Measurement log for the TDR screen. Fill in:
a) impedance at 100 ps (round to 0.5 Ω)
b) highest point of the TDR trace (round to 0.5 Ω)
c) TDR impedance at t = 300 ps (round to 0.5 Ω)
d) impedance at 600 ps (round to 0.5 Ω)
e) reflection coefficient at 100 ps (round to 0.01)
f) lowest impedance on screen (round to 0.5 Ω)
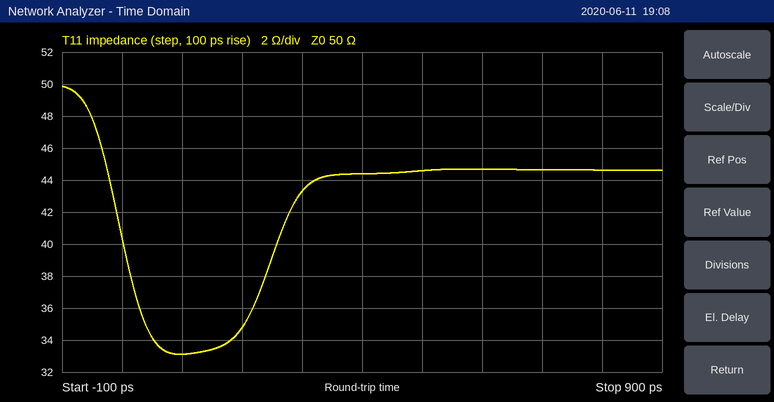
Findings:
33.0 Ω
50.0 Ω
43.5 Ω
44.5 Ω
-0.20
33.0 Ω
